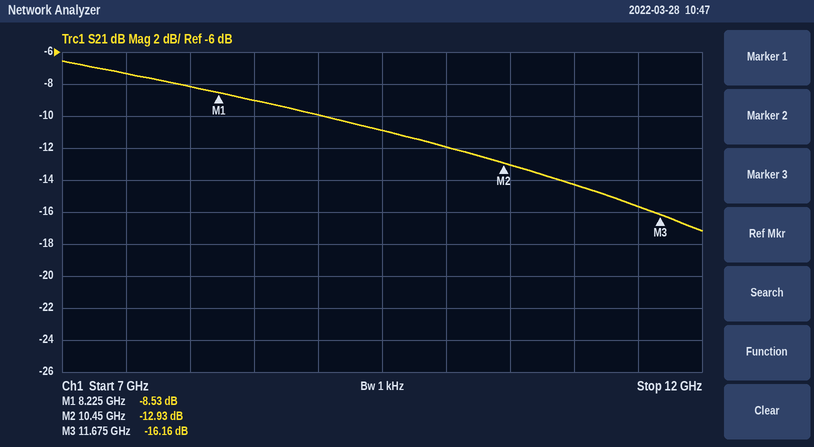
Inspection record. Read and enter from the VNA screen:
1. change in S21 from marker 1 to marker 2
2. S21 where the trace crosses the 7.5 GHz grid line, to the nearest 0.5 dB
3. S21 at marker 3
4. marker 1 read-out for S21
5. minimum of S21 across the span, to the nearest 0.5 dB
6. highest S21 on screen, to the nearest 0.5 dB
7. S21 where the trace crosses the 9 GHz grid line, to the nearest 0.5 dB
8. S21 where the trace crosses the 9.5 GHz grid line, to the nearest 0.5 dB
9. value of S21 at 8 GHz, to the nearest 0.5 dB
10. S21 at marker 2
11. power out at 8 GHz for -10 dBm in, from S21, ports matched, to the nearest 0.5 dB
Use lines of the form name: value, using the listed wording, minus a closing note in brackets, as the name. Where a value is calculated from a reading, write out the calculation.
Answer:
change in S21 from marker 1 to marker 2: -12.93 − (-8.53) = -4.40 dB
S21 where the trace crosses the 7.5 GHz grid line, to the nearest 0.5 dB: -7.5 dB
S21 at marker 3: -16.16 dB
marker 1 read-out for S21: -8.53 dB
minimum of S21 across the span, to the nearest 0.5 dB: -17.0 dB
highest S21 on screen, to the nearest 0.5 dB: -6.5 dB
S21 where the trace crosses the 9 GHz grid line, to the nearest 0.5 dB: -10.0 dB
S21 where the trace crosses the 9.5 GHz grid line, to the nearest 0.5 dB: -11.0 dB
value of S21 at 8 GHz, to the nearest 0.5 dB: -8.0 dB
S21 at marker 2: -12.93 dB
power out at 8 GHz for -10 dBm in, from S21, ports matched, to the nearest 0.5 dB: -10 dBm + (-8.0 dB) = -18.0 dBm
